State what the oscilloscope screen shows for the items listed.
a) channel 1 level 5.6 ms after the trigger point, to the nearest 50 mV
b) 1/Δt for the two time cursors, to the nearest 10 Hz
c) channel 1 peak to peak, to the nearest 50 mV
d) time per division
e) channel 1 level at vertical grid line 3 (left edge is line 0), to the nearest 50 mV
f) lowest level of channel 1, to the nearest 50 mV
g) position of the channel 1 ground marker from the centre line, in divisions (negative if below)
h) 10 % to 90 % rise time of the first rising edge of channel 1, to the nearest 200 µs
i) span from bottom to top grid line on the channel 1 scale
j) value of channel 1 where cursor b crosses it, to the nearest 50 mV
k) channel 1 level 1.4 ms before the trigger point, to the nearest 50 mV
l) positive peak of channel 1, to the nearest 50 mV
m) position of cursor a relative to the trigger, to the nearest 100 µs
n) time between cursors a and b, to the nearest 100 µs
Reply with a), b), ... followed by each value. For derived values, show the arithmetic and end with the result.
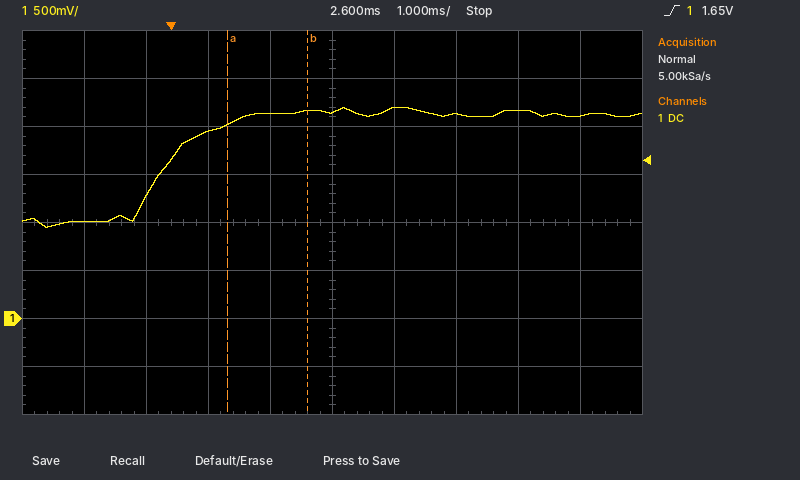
a) 2.15 V
b) 1 / 1.3 ms ≈ 770 Hz
c) 2.20 V − (950 mV) = 1.25 V
d) 1 ms
e) 1.95 V
f) 950 mV
g) -2.0 div
h) 1.4 ms
i) 4 V
j) 2.15 V
k) 1.00 V
l) 2.20 V
m) +900 µs
n) 1.3 ms
